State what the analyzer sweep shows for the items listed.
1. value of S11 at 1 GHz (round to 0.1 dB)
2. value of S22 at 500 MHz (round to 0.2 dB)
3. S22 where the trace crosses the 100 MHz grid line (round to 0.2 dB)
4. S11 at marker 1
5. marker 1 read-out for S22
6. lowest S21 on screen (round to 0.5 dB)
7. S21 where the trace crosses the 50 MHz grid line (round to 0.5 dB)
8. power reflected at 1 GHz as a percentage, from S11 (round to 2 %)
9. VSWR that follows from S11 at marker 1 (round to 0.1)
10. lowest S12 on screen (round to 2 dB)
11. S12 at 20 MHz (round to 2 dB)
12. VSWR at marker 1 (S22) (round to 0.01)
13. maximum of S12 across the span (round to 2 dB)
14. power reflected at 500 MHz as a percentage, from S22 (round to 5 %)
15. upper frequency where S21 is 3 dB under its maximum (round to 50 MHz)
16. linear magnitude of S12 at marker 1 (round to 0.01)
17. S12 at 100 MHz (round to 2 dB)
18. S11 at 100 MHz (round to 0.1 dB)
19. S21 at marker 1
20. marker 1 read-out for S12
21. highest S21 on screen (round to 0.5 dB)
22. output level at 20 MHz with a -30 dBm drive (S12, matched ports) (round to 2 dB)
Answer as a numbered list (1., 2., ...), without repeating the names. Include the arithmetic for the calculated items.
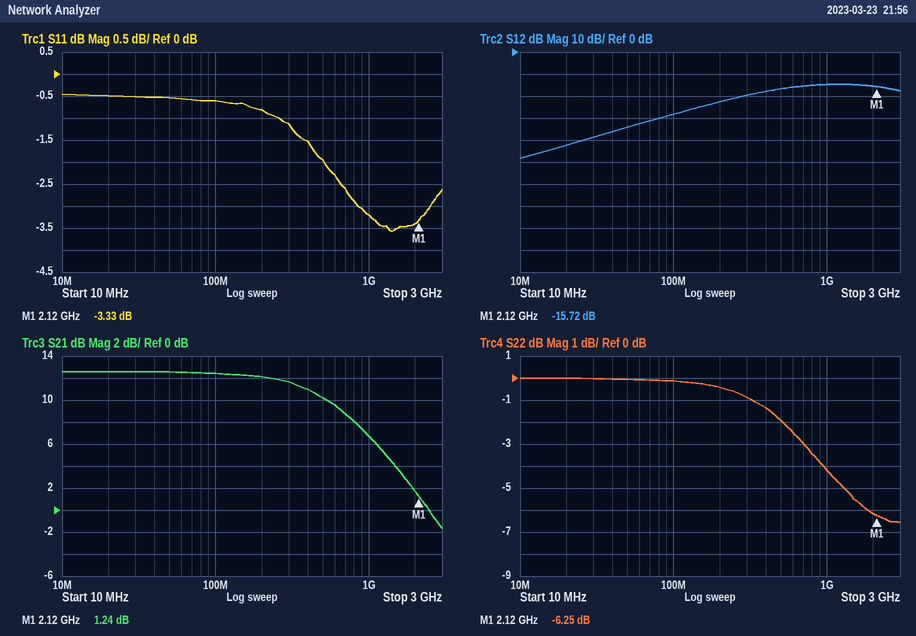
1. -3.2 dB
2. -2.0 dB
3. -0.2 dB
4. -3.33 dB
5. -6.25 dB
6. -1.5 dB
7. 12.5 dB
8. 10^(-3.2/10) ≈ 48 %
9. (1 + 0.6816)/(1 − 0.6816) ≈ 5.3
10. -48 dB
11. -42 dB
12. (1 + 0.4870)/(1 − 0.4870) ≈ 2.90
13. -14 dB
14. 10^(-2/10) ≈ 63.1 %, so 65 % to the nearest 5 %
15. 600 MHz
16. 10^(-15.72/20) ≈ 0.16
17. -28 dB
18. -0.6 dB
19. 1.24 dB
20. -15.72 dB
21. 12.5 dB
22. -30 dBm + (-42 dB) = -72 dBm
